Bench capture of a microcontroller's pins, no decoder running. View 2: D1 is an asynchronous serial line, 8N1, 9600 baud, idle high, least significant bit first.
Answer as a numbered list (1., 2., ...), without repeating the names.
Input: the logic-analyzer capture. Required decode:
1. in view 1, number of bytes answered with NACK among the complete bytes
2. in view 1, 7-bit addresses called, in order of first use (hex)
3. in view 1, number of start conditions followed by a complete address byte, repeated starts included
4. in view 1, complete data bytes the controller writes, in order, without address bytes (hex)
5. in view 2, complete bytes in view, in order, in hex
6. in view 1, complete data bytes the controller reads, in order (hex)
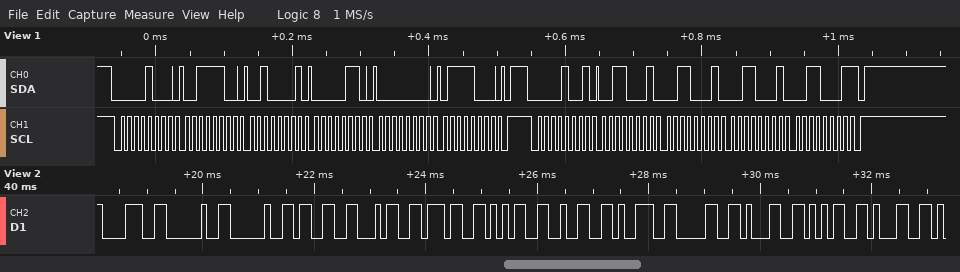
1. 1
2. 0x04
3. 2
4. 3C 21 06 00 78
5. 38 20 20 33 34 37 35 32 39 30 31 35 31
6. 31 31 31 31
